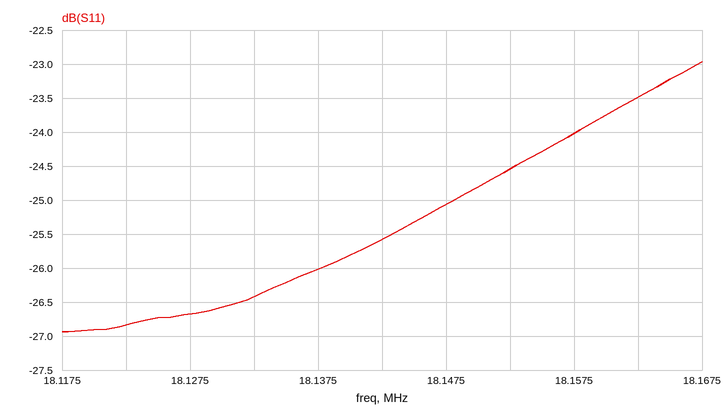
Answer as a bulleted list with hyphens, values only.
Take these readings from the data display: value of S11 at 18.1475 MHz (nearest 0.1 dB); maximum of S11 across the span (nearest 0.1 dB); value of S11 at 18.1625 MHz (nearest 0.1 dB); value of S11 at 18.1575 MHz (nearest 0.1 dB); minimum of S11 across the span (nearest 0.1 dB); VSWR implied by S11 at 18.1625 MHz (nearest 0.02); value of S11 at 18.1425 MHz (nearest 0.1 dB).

- -25.1 dB
- -23.0 dB
- -23.5 dB
- -24.0 dB
- -26.9 dB
- 1.14
- -25.6 dB
